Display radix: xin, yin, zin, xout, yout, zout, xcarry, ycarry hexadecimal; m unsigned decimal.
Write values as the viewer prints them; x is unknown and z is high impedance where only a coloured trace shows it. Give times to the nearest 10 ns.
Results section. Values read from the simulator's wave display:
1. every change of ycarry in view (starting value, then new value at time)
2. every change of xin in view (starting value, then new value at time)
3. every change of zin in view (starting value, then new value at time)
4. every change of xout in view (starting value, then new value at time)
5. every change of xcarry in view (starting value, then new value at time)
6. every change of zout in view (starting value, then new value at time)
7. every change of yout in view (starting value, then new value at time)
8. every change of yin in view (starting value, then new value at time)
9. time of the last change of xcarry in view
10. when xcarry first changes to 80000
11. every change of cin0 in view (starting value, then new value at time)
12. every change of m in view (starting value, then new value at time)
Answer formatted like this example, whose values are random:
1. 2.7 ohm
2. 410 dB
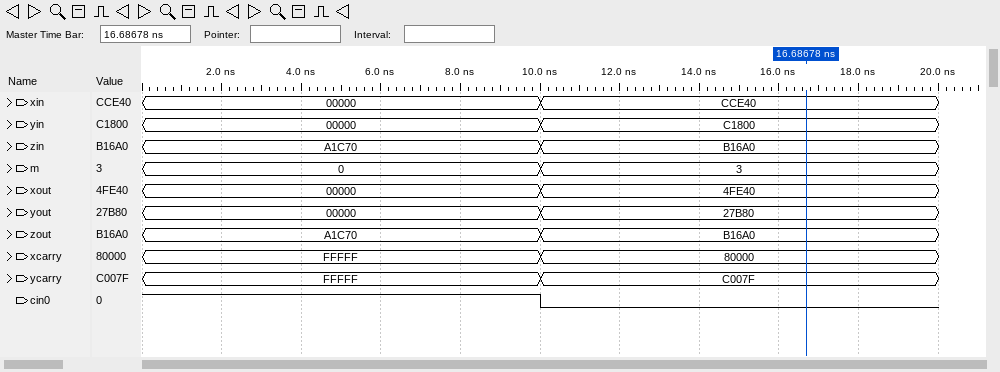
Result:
1. FFFFF, C007F at 10 ns
2. 00000, CCE40 at 10 ns
3. A1C70, B16A0 at 10 ns
4. 00000, 4FE40 at 10 ns
5. FFFFF, 80000 at 10 ns
6. A1C70, B16A0 at 10 ns
7. 00000, 27B80 at 10 ns
8. 00000, C1800 at 10 ns
9. 10 ns
10. 10 ns
11. 1, 0 at 10 ns
12. 0, 3 at 10 ns
